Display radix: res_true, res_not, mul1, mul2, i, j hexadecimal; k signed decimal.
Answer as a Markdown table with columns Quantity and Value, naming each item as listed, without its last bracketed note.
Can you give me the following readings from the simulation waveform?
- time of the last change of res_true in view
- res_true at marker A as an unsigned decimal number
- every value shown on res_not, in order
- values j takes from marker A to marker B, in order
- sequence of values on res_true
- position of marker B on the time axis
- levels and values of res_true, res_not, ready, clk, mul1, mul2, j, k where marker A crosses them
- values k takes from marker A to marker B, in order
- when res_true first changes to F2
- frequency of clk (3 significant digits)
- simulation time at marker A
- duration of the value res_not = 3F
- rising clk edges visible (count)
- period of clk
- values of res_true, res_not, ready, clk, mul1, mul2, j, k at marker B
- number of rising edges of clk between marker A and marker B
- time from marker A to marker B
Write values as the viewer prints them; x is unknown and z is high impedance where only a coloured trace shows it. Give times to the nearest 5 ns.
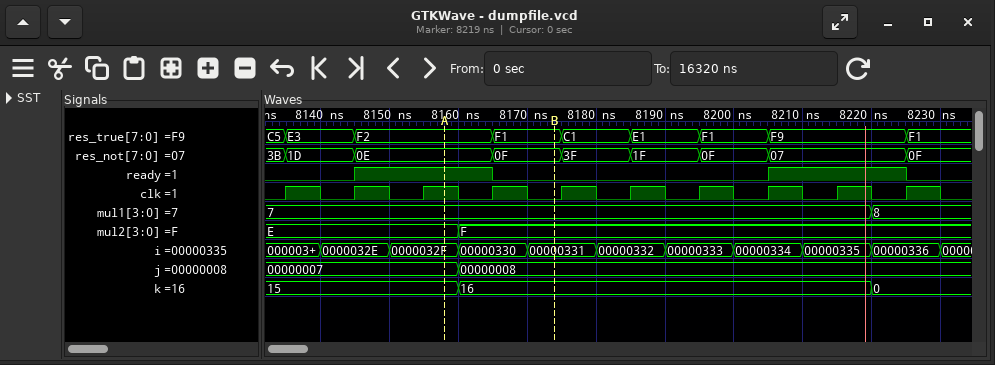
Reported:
| Quantity | Value |
|---|---|
| time of the last change of res_true in view | 8225 ns |
| res_true at marker A as an unsigned decimal number | 242 |
| every value shown on res_not, in order | 3B, 1D, 0E, 0F, 3F, 1F, 0F, 07, 0F |
| values j takes from marker A to marker B, in order | 00000007, 00000008 |
| sequence of values on res_true | C5, E3, F2, F1, C1, E1, F1, F9, F1 |
| position of marker B on the time axis | 8175 ns |
| levels and values of res_true, res_not, ready, clk, mul1, mul2, j, k where marker A crosses them | res_true=F2, res_not=0E, ready=1, clk=1, mul1=7, mul2=E, j=00000007, k=15 |
| values k takes from marker A to marker B, in order | 15, 16 |
| when res_true first changes to F2 | 8145 ns |
| frequency of clk | 100 MHz |
| simulation time at marker A | 8160 ns |
| duration of the value res_not = 3F | 10 ns |
| rising clk edges visible | 10 |
| period of clk | 10 ns |
| values of res_true, res_not, ready, clk, mul1, mul2, j, k at marker B | res_true=F1, res_not=0F, ready=0, clk=0, mul1=7, mul2=F, j=00000008, k=16 |
| number of rising edges of clk between marker A and marker B | 1 |
| time from marker A to marker B | 15 ns |
